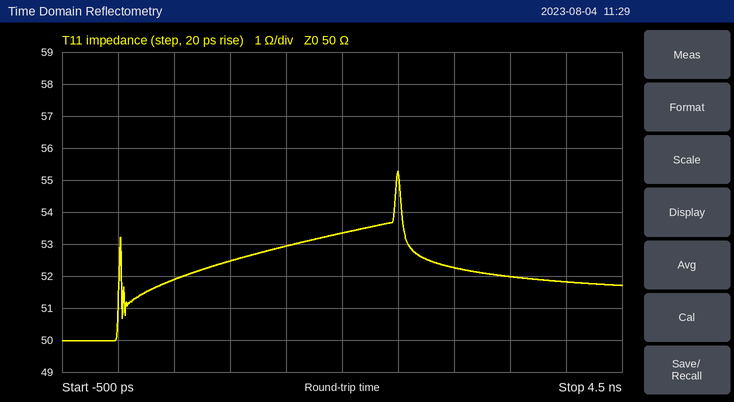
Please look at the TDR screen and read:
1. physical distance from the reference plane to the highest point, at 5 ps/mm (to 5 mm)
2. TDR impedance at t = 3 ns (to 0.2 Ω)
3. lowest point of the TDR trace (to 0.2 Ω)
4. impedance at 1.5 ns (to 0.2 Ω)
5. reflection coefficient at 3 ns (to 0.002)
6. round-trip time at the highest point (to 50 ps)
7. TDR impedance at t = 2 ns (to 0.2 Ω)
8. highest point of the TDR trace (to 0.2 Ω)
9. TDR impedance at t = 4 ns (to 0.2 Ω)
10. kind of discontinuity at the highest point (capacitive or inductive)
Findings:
250 mm
52.2 Ω
50.0 Ω
53.0 Ω
+0.022
2.50 ns
53.4 Ω
55.2 Ω
51.8 Ω
inductive
